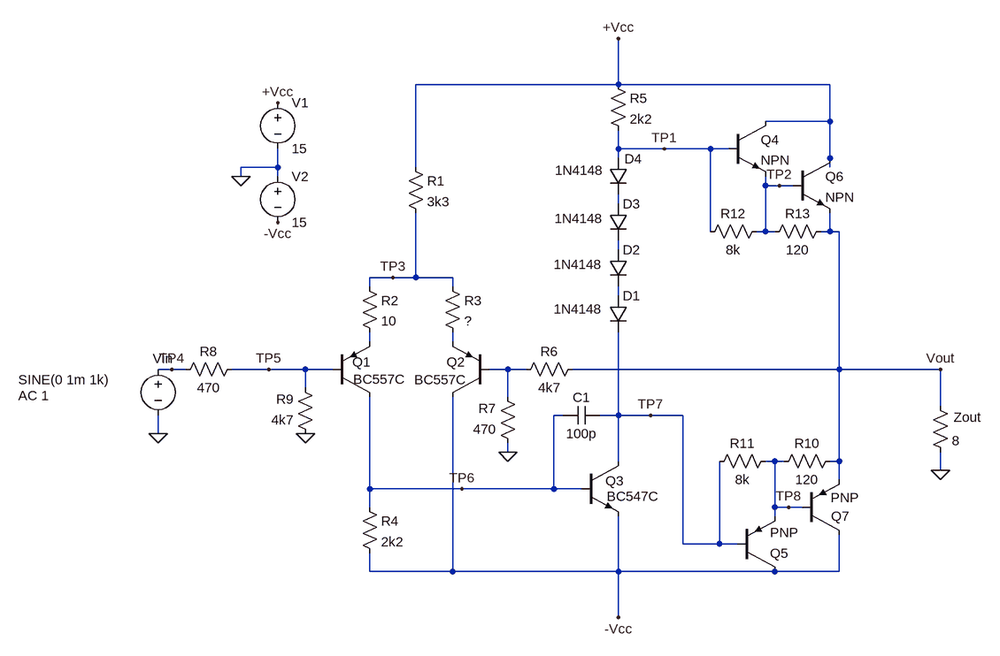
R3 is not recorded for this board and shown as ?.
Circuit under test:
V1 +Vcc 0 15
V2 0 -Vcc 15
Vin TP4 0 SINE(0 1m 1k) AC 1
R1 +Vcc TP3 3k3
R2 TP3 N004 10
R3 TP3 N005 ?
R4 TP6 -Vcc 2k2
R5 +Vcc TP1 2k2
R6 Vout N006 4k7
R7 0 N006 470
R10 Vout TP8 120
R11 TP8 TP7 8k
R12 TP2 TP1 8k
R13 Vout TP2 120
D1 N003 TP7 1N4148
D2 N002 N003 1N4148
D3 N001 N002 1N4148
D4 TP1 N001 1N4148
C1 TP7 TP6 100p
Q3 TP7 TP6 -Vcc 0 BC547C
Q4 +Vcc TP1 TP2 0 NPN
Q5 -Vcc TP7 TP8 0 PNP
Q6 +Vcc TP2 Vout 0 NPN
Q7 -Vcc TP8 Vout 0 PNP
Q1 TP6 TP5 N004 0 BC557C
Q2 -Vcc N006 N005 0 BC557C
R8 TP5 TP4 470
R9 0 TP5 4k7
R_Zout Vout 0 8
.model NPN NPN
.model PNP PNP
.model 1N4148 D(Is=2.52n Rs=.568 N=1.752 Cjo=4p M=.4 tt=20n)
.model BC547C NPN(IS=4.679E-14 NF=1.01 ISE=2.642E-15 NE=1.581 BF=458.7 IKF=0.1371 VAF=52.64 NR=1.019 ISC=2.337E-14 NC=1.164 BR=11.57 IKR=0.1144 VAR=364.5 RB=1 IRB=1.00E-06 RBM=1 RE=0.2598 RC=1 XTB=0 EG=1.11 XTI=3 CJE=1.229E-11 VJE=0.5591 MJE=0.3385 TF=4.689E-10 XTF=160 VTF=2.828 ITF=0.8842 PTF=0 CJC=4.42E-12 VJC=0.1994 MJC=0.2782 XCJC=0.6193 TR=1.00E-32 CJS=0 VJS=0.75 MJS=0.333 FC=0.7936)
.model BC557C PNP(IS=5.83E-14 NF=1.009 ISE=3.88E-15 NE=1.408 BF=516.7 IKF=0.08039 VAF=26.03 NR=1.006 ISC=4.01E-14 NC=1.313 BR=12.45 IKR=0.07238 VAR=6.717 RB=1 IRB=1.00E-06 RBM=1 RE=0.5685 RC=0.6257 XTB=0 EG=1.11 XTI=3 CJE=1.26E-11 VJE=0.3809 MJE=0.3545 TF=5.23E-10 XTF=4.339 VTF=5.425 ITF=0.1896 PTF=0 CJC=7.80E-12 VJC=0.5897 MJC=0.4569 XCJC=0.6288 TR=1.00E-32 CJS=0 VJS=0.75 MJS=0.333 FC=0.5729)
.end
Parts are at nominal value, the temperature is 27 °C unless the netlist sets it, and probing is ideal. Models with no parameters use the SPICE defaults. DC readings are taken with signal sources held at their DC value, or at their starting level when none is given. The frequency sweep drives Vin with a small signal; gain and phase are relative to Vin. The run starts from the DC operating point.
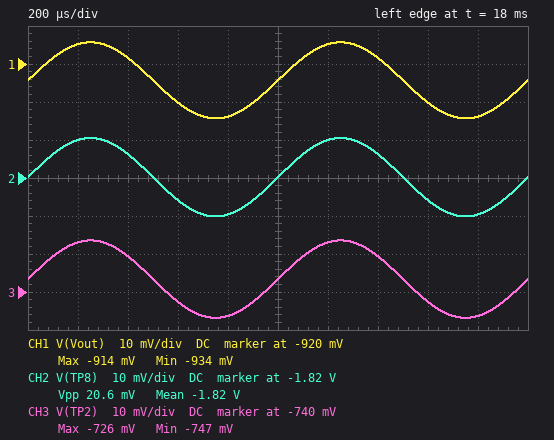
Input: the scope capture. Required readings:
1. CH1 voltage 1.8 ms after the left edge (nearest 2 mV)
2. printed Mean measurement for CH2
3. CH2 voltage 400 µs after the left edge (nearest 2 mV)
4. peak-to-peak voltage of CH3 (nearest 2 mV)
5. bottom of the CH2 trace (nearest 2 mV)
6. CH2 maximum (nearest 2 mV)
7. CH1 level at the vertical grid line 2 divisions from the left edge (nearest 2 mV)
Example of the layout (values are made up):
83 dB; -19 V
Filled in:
-934 mV; -1.82 V; -1.814 V; 20 mV; -1.830 V; -1.810 V; -918 mV
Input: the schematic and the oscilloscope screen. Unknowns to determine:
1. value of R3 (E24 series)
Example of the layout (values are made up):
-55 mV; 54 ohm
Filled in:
3.9 Ω
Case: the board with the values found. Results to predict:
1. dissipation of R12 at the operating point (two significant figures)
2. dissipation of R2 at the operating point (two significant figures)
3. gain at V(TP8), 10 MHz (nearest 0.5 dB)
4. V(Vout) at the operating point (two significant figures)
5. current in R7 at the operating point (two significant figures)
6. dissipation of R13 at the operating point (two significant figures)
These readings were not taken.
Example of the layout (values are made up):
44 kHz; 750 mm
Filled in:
77 µW; 1.0 µW; 0 dB; -920 mV; 170 µA; 290 µW
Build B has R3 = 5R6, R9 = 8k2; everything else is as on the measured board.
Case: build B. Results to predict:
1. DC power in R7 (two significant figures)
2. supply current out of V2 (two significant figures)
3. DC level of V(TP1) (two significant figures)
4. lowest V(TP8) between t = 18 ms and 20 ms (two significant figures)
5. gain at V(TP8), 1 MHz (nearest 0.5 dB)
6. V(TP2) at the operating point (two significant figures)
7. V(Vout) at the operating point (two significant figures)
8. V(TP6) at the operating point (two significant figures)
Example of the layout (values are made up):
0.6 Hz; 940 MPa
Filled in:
17 µW; 140 mA; -30 mV; -1.9 V; 19.0 dB; -810 mV; -1.0 V; -14 V
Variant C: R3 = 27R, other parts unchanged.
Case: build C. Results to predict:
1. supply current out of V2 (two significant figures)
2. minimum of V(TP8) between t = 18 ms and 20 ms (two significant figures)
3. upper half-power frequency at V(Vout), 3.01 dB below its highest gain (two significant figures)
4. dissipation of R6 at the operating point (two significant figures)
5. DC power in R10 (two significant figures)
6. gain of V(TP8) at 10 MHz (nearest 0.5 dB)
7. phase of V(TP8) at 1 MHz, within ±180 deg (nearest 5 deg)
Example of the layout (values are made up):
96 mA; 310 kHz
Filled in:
260 mA; -2.9 V; 1.2 MHz; 670 µW; 7.0 mW; -1.0 dB; -45 deg
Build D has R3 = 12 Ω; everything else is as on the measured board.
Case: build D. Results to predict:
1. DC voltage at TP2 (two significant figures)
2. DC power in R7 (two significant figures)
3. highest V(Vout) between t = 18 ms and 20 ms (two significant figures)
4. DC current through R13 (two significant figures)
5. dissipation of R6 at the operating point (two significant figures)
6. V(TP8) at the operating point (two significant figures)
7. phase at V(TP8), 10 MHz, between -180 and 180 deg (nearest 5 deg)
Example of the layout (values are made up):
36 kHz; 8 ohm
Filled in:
-1.1 V; 28 µW; -1.3 V; 1.5 mA; 290 µW; -2.2 V; -135 deg
